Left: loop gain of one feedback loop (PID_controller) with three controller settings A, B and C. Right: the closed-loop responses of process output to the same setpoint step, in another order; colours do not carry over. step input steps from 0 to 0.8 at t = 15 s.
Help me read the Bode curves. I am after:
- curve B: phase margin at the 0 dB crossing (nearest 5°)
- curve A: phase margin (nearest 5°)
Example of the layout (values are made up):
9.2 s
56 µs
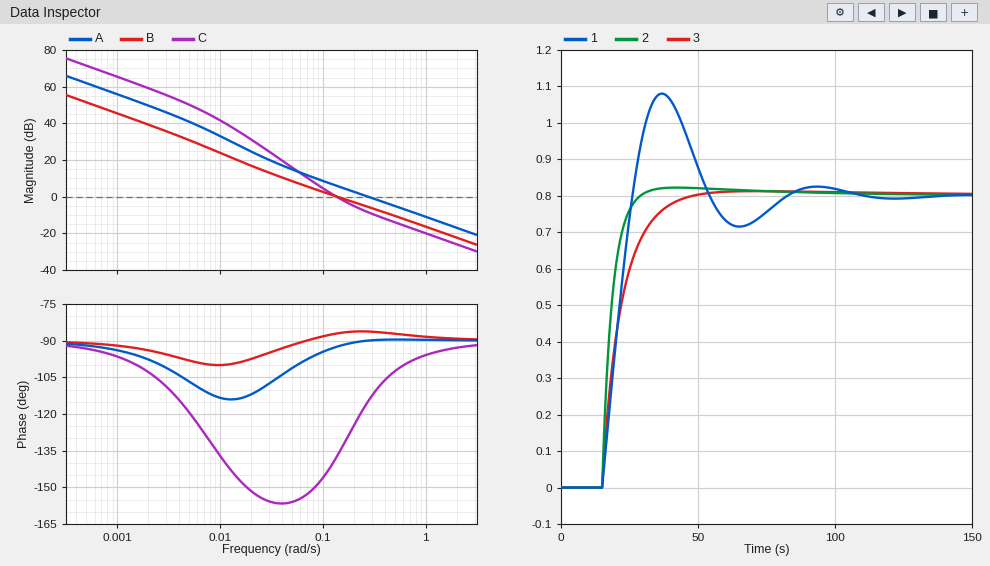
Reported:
95°
90°
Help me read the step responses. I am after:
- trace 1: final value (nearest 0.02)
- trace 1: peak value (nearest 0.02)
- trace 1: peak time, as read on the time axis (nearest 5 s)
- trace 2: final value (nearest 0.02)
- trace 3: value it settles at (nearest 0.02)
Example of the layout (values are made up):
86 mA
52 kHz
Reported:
0.80
1.08
35 s
0.80
0.80
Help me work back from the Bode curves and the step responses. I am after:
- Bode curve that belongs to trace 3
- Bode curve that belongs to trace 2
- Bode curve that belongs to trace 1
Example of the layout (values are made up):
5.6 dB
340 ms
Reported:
B
A
C
